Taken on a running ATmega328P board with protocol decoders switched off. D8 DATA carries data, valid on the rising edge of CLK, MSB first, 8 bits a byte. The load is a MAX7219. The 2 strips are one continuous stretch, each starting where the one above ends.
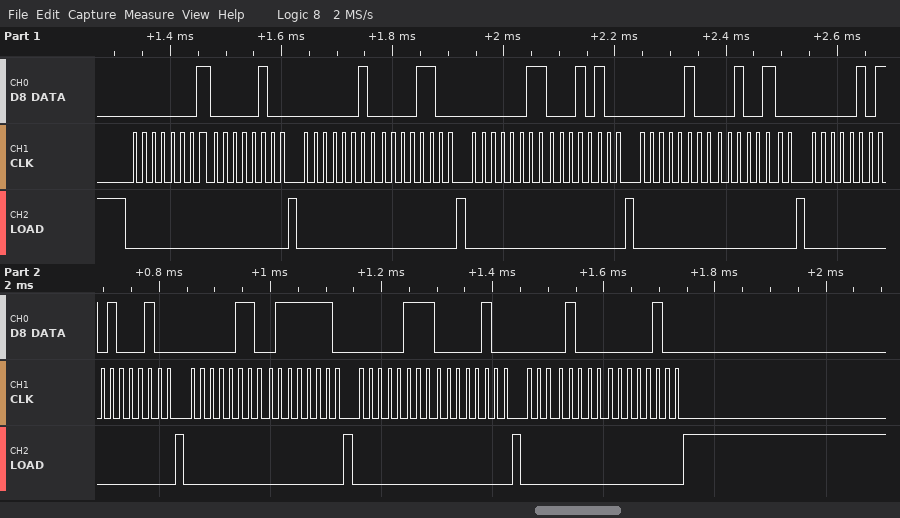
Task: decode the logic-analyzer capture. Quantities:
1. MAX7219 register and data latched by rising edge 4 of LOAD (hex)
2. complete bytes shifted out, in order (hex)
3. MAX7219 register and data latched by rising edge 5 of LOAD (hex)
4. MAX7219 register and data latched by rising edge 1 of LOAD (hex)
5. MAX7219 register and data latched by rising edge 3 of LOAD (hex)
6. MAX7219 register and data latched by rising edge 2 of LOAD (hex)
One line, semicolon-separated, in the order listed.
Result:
register 0x4, data 0x24; 01 04 02 0C 03 14 04 24 05 44 06 7E 07 04 08 04; register 0x5, data 0x44; register 0x1, data 0x04; register 0x3, data 0x14; register 0x2, data 0x0C
